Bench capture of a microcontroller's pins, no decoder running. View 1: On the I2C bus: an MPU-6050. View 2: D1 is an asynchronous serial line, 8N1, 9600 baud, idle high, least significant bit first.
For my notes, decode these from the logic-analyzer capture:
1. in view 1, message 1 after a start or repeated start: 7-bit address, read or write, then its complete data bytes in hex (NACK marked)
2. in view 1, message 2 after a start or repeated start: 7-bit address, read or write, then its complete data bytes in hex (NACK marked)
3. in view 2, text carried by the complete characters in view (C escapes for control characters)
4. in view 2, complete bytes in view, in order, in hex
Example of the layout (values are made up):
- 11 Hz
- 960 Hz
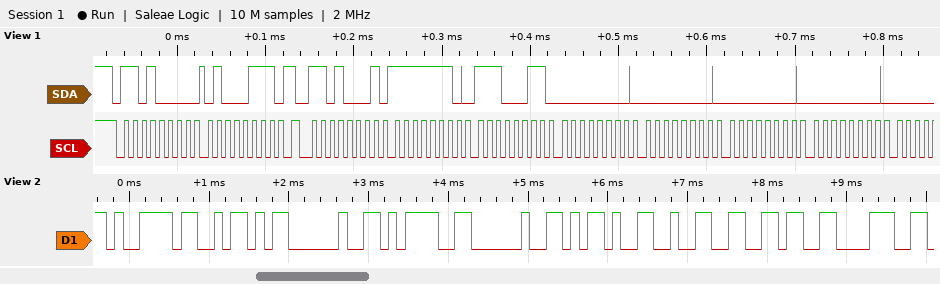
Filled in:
- 0x68 write: 47
- 0x68 read: FE E3 00 00 00 00
- "yZ = -268"
- 79 5A 20 3D 20 2D 32 36 38
